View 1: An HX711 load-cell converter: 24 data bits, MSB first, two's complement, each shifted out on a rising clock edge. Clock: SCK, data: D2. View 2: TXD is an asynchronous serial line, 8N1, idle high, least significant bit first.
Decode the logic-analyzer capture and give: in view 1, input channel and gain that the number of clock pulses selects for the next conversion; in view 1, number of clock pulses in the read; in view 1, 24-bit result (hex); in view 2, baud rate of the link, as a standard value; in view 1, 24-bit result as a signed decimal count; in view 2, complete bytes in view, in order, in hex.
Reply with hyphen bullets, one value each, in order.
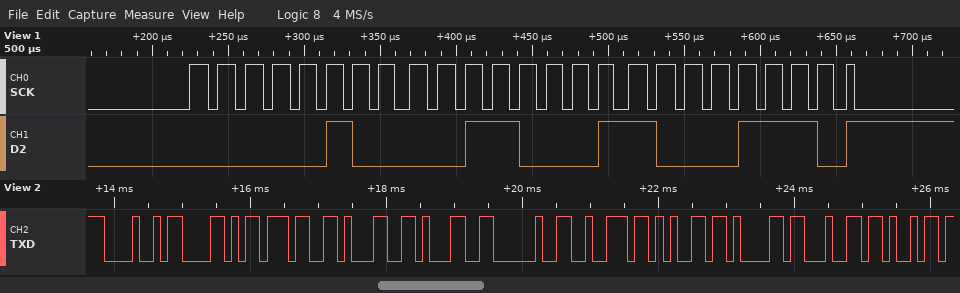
- channel A, gain 128
- 25
- 0x04318E
- 9600 baud
- 274830
- 0x48 0x58 0x37 0x31 0x31 0x20 0x72 0x65 0x61 0x64 0x69
